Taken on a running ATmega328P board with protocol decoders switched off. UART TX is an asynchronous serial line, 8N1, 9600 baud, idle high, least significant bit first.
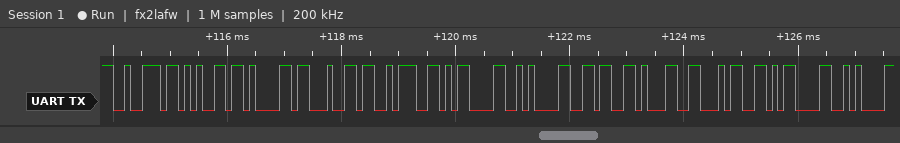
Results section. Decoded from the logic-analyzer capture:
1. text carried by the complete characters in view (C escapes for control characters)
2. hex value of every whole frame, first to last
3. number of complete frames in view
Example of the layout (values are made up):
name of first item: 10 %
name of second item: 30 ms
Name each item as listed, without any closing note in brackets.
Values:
text carried by the complete characters in view: "read:\r\n614\r\n"
hex value of every whole frame, first to last: 0x72 0x65 0x61 0x64 0x3A 0x0D 0x0A 0x36 0x31 0x34 0x0D 0x0A
number of complete frames in view: 12
